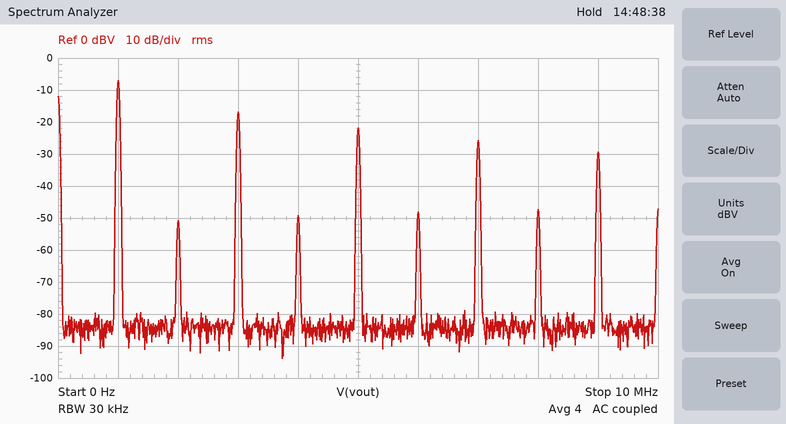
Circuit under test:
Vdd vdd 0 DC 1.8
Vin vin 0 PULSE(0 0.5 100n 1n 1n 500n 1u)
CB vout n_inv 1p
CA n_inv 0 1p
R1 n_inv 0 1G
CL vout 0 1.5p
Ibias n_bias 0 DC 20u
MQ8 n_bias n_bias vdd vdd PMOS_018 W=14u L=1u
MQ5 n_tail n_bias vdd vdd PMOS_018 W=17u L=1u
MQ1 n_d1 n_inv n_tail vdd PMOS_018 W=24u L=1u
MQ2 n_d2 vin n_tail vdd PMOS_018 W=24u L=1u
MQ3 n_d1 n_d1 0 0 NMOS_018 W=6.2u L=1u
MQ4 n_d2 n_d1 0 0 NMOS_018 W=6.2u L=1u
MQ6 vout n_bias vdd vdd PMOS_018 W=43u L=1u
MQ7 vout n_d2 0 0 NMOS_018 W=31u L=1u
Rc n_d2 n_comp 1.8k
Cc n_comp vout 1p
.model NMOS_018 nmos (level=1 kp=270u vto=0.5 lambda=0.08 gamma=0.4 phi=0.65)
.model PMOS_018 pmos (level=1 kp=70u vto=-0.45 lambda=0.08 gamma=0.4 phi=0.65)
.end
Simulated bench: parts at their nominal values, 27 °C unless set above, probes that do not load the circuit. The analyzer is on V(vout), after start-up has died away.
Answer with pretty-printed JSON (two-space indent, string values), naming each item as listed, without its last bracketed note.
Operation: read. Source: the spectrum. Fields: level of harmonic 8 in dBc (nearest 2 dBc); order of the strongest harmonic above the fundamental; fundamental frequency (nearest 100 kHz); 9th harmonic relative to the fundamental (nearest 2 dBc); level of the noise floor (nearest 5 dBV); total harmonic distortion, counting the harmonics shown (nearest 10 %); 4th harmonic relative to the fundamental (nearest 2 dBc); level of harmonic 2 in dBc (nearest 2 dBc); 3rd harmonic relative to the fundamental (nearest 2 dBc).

{
  "level of harmonic 8 in dBc": "-40 dBc",
  "order of the strongest harmonic above the fundamental": "3",
  "fundamental frequency": "1.0 MHz",
  "9th harmonic relative to the fundamental": "-22 dBc",
  "level of the noise floor": "-85 dBV",
  "total harmonic distortion, counting the harmonics shown": "40 %",
  "4th harmonic relative to the fundamental": "-42 dBc",
  "level of harmonic 2 in dBc": "-44 dBc",
  "3rd harmonic relative to the fundamental": "-10 dBc"
}
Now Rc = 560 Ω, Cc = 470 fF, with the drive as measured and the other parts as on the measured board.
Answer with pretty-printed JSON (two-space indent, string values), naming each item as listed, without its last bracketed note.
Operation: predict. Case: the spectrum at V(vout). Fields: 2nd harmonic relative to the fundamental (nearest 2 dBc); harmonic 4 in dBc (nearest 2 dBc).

{
  "2nd harmonic relative to the fundamental": "-30 dBc",
  "harmonic 4 in dBc": "-30 dBc"
}
